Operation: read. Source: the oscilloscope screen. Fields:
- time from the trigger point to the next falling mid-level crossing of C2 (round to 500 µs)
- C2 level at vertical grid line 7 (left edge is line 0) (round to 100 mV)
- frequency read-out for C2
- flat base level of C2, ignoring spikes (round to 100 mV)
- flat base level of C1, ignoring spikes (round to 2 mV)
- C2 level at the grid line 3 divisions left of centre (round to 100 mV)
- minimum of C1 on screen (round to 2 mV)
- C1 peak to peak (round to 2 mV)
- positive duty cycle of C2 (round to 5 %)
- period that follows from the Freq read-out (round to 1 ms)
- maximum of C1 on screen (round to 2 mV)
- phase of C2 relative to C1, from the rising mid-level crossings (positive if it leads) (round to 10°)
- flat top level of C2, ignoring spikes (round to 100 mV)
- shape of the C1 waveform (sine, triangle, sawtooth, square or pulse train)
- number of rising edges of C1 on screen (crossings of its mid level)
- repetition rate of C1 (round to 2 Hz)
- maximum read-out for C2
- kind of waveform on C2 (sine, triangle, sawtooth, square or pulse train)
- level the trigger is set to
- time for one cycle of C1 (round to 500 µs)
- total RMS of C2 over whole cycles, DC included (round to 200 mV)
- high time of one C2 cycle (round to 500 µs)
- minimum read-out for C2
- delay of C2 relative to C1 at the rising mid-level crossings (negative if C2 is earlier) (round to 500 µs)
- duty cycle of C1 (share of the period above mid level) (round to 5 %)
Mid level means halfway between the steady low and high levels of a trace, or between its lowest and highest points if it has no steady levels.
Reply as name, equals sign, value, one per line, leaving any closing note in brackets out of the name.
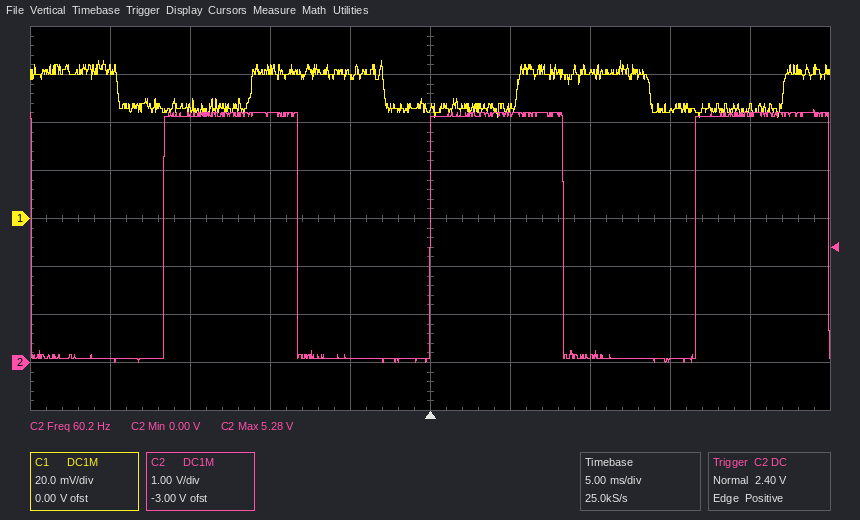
time from the trigger point to the next falling mid-level crossing of C2 = 8.5 ms
C2 level at vertical grid line 7 (left edge is line 0) = 100 mV
frequency read-out for C2 = 60.2 Hz
flat base level of C2, ignoring spikes = 100 mV
flat base level of C1, ignoring spikes = 46 mV
C2 level at the grid line 3 divisions left of centre = 5.2 V
minimum of C1 on screen = 42 mV
C1 peak to peak = 24 mV
positive duty cycle of C2 = 50 %
period that follows from the Freq read-out = 17 ms
maximum of C1 on screen = 66 mV
phase of C2 relative to C1, from the rising mid-level crossings (positive if it leads) = +120°
flat top level of C2, ignoring spikes = 5.2 V
shape of the C1 waveform = square
number of rising edges of C1 on screen = 3
repetition rate of C1 = 60 Hz
maximum read-out for C2 = 5.28 V
kind of waveform on C2 = square
level the trigger is set to = 2.40 V
time for one cycle of C1 = 16.5 ms
total RMS of C2 over whole cycles, DC included = 3.6 V
high time of one C2 cycle = 8.5 ms
minimum read-out for C2 = 0.00 V
delay of C2 relative to C1 at the rising mid-level crossings (negative if C2 is earlier) = -5.5 ms
duty cycle of C1 (share of the period above mid level) = 50 %
